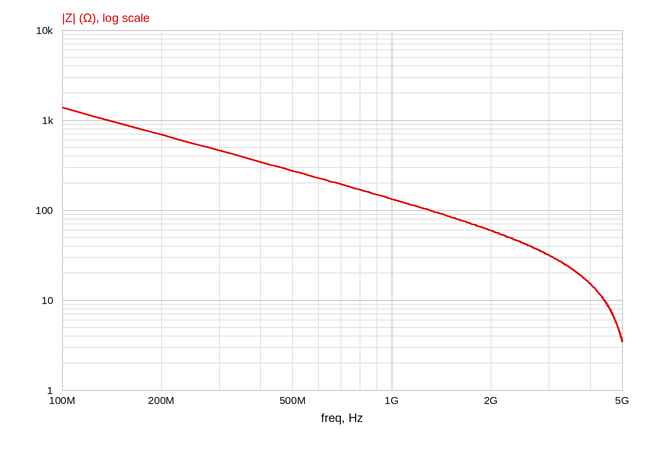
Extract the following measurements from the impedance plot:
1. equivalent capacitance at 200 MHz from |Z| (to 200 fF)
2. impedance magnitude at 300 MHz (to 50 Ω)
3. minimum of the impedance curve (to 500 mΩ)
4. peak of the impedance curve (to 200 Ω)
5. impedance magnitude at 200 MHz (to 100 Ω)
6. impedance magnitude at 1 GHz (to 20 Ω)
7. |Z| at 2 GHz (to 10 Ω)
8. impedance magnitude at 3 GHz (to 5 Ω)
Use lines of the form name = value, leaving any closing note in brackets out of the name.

equivalent capacitance at 200 MHz from |Z| = 1.2 pF
impedance magnitude at 300 MHz = 450 Ω
minimum of the impedance curve = 3.5 Ω
peak of the impedance curve = 1.4 kΩ
impedance magnitude at 200 MHz = 700 Ω
impedance magnitude at 1 GHz = 140 Ω
|Z| at 2 GHz = 60 Ω
impedance magnitude at 3 GHz = 30 Ω
